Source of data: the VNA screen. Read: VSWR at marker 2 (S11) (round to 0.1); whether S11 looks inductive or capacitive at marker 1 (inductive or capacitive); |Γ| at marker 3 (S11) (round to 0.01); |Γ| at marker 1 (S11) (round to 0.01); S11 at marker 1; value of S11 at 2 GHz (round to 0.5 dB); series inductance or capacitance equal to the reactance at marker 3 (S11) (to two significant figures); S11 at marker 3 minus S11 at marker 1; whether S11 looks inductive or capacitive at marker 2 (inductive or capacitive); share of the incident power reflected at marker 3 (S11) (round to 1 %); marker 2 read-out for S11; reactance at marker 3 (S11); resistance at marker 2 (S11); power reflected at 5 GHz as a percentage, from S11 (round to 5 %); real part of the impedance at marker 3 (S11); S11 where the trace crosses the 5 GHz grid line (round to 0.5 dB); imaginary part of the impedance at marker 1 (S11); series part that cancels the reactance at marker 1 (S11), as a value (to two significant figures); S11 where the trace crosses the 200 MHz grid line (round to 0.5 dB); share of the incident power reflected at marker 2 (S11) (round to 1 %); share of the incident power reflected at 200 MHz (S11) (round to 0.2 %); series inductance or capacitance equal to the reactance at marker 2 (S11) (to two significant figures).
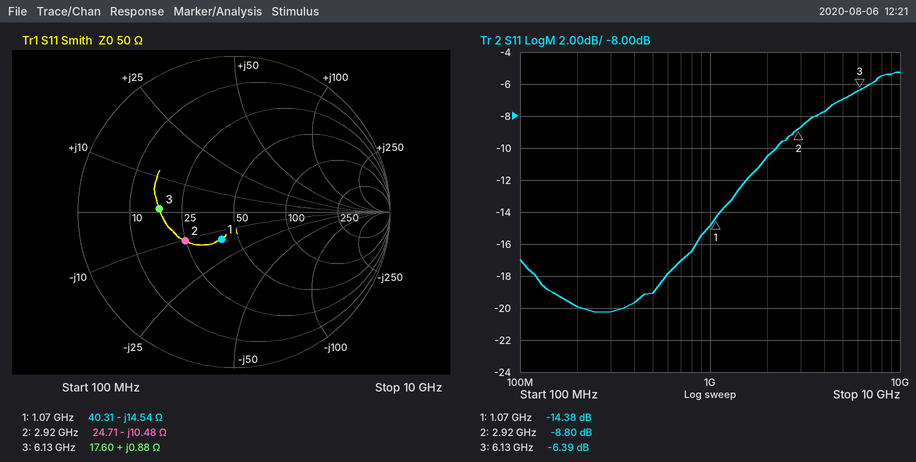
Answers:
2.1
capacitive
0.48
0.19
-14.38 dB
-10.5 dB
23 pH
7.99 dB
capacitive
23 %
-8.80 dB
+0.88 Ω
24.71 Ω
20 %
17.60 Ω
-7.0 dB
-14.54 Ω
2.2 nH
-20.0 dB
13 %
1.0 %
5.2 pF
